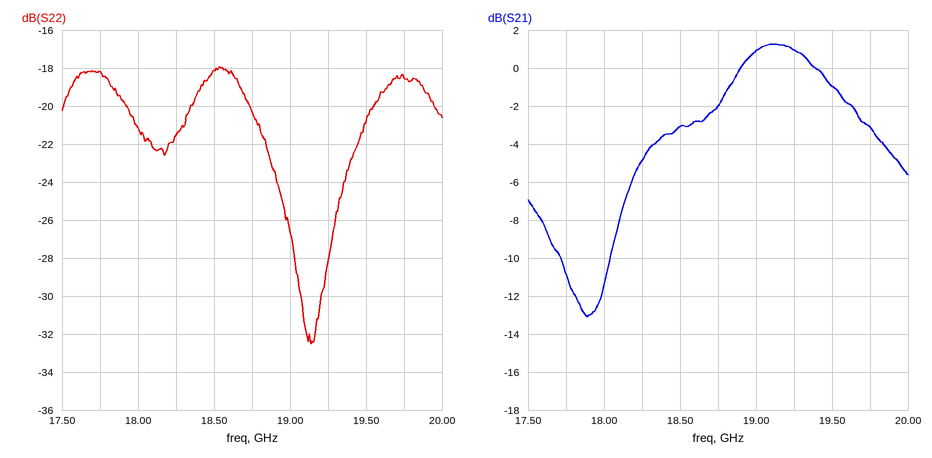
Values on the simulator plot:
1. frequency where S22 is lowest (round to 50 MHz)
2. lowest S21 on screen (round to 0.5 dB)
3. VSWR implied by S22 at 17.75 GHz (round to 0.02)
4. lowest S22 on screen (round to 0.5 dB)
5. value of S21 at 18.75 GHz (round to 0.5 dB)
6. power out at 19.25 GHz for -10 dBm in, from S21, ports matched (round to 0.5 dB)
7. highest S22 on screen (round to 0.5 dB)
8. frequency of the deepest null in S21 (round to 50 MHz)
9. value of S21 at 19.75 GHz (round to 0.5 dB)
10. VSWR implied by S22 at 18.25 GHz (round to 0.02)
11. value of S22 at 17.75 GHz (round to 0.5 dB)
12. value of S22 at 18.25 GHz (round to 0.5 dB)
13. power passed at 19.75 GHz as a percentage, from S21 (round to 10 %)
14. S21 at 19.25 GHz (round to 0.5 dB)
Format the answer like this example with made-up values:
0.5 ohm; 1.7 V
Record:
19.15 GHz; -13.0 dB; 1.28; -32.5 dB; -2.0 dB; -9.0 dBm; -18.0 dB; 17.90 GHz; -3.0 dB; 1.18; -18.0 dB; -21.5 dB; 50 %; 1.0 dB
